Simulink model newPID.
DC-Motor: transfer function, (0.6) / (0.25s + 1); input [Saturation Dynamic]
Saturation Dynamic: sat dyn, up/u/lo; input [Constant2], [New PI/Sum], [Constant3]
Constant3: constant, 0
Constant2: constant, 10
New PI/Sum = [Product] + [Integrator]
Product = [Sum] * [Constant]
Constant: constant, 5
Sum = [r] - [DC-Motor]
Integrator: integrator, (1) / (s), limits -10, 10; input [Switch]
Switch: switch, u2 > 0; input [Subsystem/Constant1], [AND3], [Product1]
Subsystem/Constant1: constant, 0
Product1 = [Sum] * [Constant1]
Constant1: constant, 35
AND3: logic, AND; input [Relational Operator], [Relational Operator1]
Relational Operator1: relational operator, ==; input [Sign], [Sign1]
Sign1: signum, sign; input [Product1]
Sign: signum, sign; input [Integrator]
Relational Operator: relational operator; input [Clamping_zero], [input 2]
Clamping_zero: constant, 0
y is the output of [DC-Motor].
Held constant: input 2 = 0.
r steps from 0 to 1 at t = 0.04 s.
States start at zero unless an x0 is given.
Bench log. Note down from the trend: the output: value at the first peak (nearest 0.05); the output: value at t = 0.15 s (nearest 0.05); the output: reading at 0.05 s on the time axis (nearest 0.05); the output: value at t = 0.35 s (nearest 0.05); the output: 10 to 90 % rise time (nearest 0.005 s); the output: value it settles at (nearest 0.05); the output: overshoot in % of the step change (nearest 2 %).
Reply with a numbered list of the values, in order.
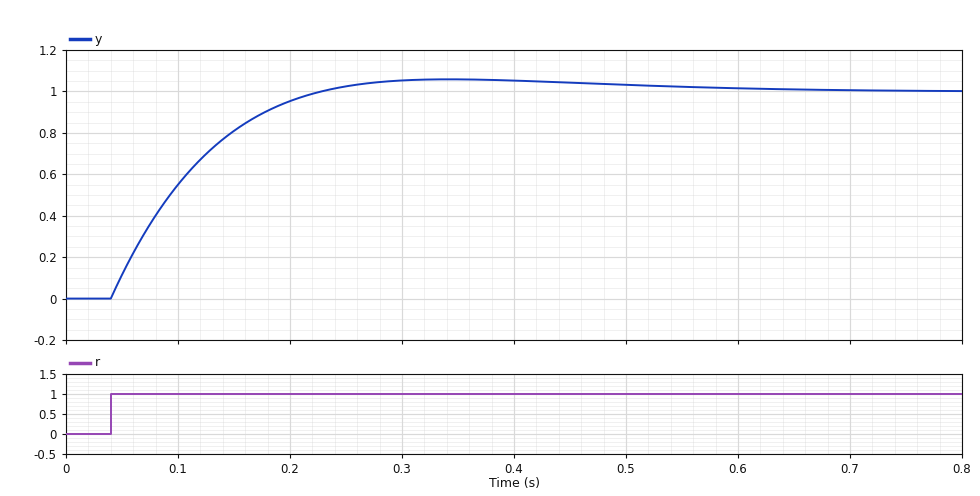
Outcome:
1. 1.05
2. 0.80
3. 0.10
4. 1.05
5. 0.130 s
6. 1.00
7. 6 %
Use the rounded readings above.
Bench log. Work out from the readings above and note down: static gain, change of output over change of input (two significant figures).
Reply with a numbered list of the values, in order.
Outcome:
1. 1.0
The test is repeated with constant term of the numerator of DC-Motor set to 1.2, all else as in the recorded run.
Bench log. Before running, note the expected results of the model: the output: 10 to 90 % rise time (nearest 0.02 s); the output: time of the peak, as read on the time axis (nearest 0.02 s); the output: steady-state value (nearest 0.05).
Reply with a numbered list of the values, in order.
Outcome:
1. 0.08 s
2. 0.22 s
3. 1.00
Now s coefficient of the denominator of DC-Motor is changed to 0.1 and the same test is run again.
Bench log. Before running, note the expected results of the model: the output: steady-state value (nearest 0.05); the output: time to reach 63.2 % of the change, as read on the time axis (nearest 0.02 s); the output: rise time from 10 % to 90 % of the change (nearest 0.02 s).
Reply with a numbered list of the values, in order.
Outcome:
1. 1.00
2. 0.08 s
3. 0.10 s
